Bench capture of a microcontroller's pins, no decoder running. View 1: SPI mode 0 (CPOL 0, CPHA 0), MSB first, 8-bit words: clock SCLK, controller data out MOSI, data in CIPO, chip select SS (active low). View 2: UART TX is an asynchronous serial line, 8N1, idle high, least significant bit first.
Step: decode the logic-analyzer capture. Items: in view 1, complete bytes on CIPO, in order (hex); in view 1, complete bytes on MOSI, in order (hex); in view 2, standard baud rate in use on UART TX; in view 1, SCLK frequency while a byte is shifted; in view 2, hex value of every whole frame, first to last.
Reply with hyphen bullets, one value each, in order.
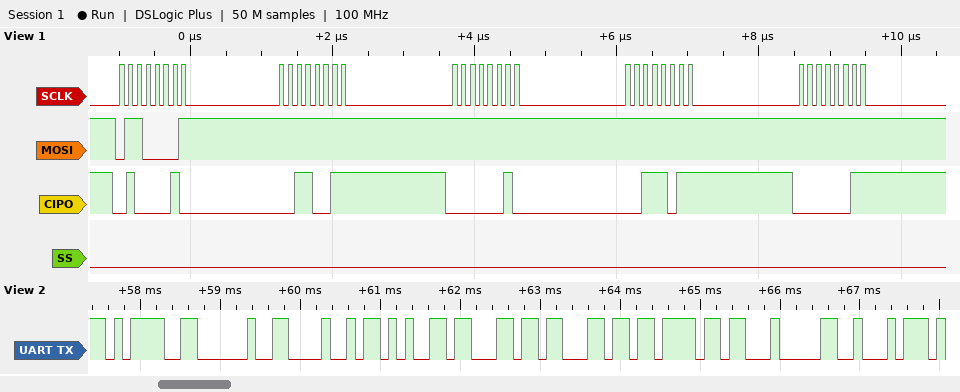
- 42 33 02 3B 03
- 61 FF FF FF FF
- 9600 baud
- 8 MHz
- 3D 20 48 65 6C 6C 6F 04 A2
